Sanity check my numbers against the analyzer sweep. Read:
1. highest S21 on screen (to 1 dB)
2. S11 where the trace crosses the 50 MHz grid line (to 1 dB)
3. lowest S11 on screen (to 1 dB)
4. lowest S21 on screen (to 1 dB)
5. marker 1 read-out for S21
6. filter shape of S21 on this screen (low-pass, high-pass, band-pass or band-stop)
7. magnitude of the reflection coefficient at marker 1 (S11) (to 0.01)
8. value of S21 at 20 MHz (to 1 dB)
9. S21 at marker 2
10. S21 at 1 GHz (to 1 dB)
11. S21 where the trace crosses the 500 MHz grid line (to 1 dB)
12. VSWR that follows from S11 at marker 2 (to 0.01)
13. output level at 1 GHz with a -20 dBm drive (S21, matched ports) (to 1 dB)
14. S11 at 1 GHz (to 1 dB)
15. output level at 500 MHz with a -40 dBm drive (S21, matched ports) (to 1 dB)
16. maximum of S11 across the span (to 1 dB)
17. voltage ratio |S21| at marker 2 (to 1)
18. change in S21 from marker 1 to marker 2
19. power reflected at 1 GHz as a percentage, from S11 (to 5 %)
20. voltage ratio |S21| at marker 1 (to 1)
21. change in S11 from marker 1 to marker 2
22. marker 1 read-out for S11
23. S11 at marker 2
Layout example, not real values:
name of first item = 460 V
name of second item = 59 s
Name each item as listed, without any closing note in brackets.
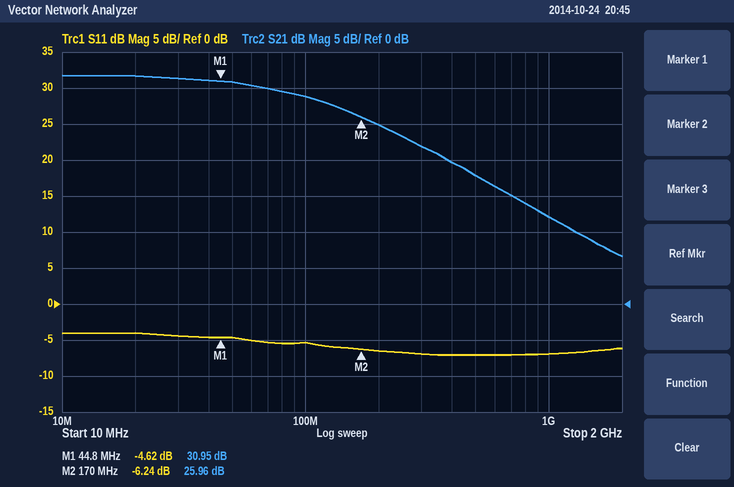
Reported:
highest S21 on screen = 32 dB
S11 where the trace crosses the 50 MHz grid line = -5 dB
lowest S11 on screen = -7 dB
lowest S21 on screen = 7 dB
marker 1 read-out for S21 = 30.95 dB
filter shape of S21 on this screen = low-pass
magnitude of the reflection coefficient at marker 1 (S11) = 0.59
value of S21 at 20 MHz = 32 dB
S21 at marker 2 = 25.96 dB
S21 at 1 GHz = 12 dB
S21 where the trace crosses the 500 MHz grid line = 18 dB
VSWR that follows from S11 at marker 2 = 2.90
output level at 1 GHz with a -20 dBm drive (S21, matched ports) = -8 dBm
S11 at 1 GHz = -7 dB
output level at 500 MHz with a -40 dBm drive (S21, matched ports) = -22 dBm
maximum of S11 across the span = -4 dB
voltage ratio |S21| at marker 2 = 20
change in S21 from marker 1 to marker 2 = -4.99 dB
power reflected at 1 GHz as a percentage, from S11 = 20 %
voltage ratio |S21| at marker 1 = 35
change in S11 from marker 1 to marker 2 = -1.62 dB
marker 1 read-out for S11 = -4.62 dB
S11 at marker 2 = -6.24 dB
